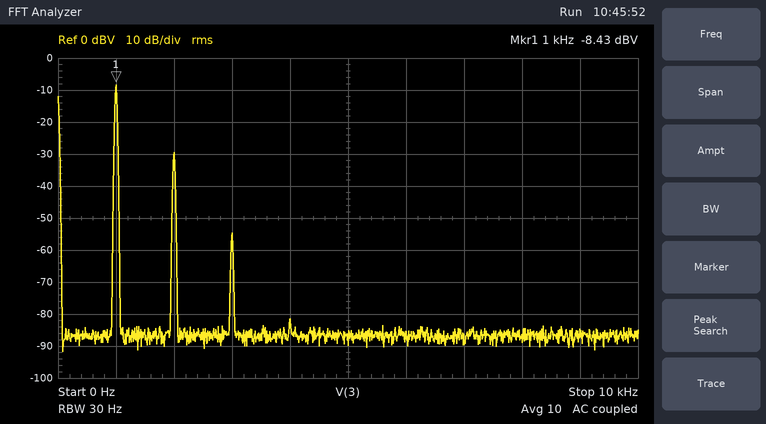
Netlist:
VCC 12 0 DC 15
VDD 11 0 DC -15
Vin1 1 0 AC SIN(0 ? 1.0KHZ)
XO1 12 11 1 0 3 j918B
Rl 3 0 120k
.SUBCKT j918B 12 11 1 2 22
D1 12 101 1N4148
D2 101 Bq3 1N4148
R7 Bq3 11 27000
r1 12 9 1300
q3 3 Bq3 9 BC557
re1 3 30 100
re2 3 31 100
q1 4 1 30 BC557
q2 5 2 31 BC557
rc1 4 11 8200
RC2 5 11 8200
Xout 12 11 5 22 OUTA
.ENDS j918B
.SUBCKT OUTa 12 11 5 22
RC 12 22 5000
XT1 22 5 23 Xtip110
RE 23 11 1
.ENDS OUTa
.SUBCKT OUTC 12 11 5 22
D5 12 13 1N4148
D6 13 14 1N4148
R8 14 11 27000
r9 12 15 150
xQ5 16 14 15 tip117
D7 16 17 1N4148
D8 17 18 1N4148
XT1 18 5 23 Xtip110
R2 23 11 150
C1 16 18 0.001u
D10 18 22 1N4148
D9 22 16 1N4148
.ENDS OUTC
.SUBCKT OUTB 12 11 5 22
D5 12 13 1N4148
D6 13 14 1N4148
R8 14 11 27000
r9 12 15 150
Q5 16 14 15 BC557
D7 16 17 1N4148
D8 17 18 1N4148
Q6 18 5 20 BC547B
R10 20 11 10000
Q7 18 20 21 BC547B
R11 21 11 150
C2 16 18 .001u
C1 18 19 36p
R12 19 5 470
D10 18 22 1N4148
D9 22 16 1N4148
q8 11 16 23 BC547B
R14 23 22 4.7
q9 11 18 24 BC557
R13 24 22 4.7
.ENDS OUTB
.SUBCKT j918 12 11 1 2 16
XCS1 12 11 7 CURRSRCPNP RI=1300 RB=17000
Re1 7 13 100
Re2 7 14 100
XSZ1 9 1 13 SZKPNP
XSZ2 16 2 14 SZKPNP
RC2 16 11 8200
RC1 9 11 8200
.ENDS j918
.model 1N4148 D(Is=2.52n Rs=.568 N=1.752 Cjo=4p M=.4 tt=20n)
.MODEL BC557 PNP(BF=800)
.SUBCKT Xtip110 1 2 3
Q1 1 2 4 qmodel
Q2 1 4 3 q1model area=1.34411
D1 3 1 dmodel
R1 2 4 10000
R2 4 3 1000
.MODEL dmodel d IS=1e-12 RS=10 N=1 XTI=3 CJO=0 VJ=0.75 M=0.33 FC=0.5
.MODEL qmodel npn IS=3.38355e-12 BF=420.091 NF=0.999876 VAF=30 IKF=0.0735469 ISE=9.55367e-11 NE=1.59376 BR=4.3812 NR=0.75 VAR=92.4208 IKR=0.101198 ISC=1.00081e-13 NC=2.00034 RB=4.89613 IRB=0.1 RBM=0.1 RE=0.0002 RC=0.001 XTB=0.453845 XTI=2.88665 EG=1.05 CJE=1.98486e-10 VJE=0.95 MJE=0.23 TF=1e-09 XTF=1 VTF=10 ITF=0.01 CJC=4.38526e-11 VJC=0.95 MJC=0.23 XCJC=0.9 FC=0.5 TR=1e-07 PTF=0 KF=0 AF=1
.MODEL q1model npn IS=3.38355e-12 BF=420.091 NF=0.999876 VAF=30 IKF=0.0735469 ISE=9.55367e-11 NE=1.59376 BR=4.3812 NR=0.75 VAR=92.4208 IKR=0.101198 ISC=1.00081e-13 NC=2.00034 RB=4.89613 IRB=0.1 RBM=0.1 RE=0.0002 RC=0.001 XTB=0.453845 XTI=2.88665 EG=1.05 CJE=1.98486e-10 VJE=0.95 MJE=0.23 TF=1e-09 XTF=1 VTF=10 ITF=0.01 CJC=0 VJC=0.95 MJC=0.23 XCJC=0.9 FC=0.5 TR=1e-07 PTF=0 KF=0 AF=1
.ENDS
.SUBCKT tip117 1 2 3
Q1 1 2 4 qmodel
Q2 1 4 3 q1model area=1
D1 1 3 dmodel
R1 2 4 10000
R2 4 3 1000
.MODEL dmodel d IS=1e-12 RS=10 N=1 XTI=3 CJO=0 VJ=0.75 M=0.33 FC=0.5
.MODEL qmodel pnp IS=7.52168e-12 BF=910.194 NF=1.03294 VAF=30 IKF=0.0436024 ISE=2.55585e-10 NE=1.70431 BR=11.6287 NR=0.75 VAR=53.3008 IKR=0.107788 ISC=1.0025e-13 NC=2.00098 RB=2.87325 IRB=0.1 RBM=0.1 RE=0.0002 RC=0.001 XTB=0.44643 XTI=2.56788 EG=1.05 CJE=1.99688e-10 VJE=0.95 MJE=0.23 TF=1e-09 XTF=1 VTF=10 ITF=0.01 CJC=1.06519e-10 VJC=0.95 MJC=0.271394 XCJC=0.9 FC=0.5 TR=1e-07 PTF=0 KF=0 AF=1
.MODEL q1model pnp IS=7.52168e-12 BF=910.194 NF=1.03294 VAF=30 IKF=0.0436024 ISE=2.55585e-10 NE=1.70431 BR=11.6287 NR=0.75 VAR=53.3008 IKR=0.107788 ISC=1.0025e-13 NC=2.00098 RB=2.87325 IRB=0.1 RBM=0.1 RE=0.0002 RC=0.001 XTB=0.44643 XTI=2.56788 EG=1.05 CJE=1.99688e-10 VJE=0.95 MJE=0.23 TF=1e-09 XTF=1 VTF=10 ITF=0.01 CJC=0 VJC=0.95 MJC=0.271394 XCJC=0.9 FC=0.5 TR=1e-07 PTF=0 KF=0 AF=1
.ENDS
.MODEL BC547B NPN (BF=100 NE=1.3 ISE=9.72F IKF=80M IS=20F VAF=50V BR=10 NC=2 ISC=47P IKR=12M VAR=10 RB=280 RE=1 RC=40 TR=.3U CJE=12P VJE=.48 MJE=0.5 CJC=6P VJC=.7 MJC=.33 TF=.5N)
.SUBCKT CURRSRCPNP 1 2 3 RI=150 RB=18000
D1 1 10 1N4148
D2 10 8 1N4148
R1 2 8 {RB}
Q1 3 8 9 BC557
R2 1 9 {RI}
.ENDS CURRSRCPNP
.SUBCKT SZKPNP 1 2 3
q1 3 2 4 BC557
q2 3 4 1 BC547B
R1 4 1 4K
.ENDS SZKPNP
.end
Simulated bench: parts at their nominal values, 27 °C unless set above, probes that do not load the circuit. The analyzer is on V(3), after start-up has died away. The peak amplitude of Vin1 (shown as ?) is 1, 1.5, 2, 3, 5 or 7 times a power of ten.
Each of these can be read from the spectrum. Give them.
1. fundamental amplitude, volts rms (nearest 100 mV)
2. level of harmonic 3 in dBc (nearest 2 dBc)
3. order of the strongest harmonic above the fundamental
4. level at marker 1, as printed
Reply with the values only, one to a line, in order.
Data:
400 mV
-46 dBc
2
-8.43 dBV
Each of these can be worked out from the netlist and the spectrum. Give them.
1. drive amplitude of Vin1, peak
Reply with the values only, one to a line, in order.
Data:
1 mV
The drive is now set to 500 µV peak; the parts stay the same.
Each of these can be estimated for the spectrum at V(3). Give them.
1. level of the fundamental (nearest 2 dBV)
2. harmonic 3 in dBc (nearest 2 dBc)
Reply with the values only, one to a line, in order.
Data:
-14 dBV
-58 dBc
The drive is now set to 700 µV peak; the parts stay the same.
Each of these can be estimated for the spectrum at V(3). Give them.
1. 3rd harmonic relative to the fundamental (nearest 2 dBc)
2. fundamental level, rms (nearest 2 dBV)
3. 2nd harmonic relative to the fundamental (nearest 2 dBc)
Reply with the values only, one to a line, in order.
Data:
-52 dBc
-12 dBV
-24 dBc
